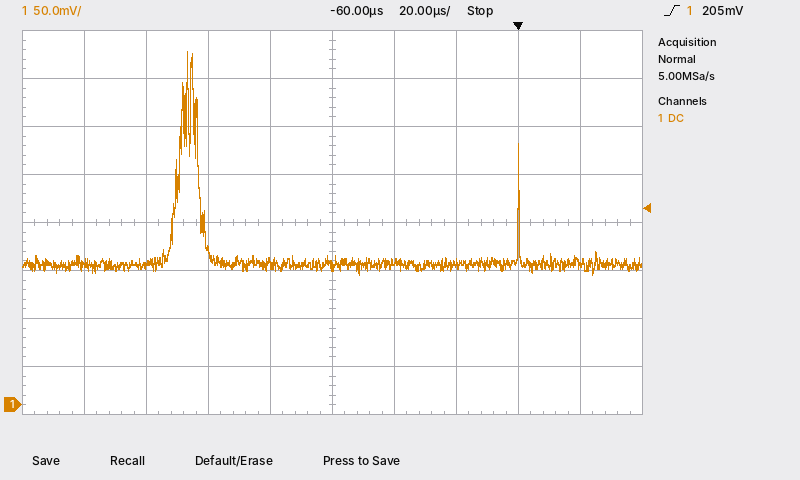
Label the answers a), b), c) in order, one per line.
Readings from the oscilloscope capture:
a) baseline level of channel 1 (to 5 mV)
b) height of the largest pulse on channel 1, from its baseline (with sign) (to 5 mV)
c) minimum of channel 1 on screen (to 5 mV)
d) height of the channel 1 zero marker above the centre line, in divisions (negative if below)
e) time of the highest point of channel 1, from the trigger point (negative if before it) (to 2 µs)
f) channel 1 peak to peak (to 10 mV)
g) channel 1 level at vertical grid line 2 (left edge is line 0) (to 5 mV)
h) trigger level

a) 145 mV
b) +220 mV
c) 135 mV
d) -3.8 div
e) -106 µs
f) 230 mV
g) 145 mV
h) 205 mV
